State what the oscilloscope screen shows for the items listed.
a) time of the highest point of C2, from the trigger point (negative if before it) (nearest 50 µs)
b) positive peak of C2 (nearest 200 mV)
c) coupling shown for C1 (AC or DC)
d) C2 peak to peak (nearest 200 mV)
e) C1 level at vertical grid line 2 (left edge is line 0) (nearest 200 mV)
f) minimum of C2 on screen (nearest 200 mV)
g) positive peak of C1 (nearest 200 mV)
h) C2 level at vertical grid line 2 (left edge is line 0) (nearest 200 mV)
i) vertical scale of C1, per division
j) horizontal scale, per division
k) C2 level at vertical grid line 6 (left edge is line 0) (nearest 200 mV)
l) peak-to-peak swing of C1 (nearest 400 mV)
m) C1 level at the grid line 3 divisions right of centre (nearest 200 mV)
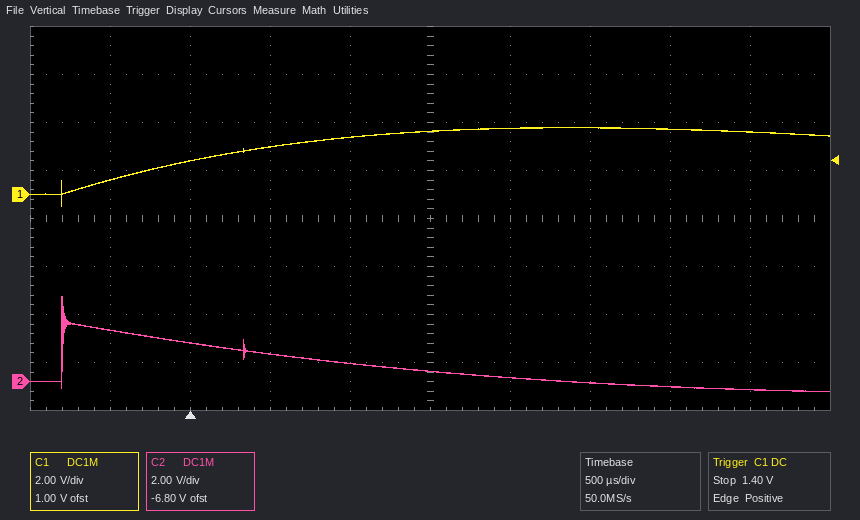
-800 µs
3.6 V
DC
4.0 V
1.4 V
-400 mV
2.8 V
1.6 V
2 V
500 µs
200 mV
3.2 V
2.8 V
